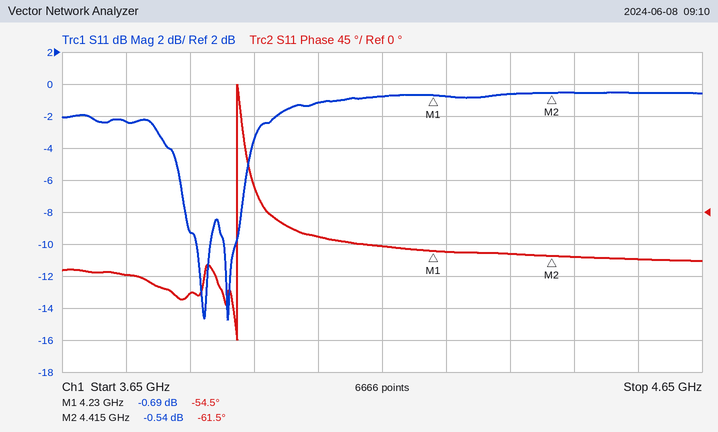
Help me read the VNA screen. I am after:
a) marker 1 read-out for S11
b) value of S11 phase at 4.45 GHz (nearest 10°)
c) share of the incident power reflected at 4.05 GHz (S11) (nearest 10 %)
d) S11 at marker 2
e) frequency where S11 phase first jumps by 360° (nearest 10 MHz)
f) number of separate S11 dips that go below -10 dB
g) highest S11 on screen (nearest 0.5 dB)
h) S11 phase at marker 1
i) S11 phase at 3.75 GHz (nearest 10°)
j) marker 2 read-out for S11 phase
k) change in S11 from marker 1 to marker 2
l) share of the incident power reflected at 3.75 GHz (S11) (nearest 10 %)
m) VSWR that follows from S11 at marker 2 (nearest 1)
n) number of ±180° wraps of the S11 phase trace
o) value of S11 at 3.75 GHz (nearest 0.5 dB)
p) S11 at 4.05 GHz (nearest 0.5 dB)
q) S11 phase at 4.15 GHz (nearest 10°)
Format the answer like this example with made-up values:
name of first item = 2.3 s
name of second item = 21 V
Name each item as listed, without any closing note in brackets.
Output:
marker 1 read-out for S11 = -0.69 dB
value of S11 phase at 4.45 GHz = -60°
share of the incident power reflected at 4.05 GHz (S11) = 80 %
S11 at marker 2 = -0.54 dB
frequency where S11 phase first jumps by 360° = 3.92 GHz
number of separate S11 dips that go below -10 dB = 2
highest S11 on screen = -0.5 dB
S11 phase at marker 1 = -54.5°
S11 phase at 3.75 GHz = -90°
marker 2 read-out for S11 phase = -61.5°
change in S11 from marker 1 to marker 2 = 0.15 dB
share of the incident power reflected at 3.75 GHz (S11) = 60 %
VSWR that follows from S11 at marker 2 = 32
number of ±180° wraps of the S11 phase trace = 1
value of S11 at 3.75 GHz = -2.5 dB
S11 at 4.05 GHz = -1.0 dB
S11 phase at 4.15 GHz = -50°
